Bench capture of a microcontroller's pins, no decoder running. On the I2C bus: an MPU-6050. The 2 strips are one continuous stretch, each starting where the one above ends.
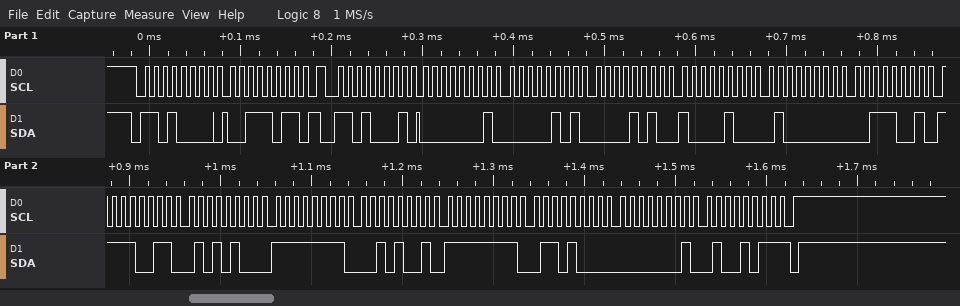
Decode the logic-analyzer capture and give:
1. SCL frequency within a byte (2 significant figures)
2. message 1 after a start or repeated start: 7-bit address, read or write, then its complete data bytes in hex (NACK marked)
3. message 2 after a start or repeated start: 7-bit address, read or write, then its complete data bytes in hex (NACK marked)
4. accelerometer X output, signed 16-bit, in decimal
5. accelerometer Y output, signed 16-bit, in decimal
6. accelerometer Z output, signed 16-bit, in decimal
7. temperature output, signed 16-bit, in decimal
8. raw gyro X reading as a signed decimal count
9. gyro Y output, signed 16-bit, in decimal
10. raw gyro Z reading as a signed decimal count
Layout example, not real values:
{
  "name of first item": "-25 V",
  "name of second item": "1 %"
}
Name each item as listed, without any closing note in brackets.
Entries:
{
  "SCL frequency within a byte": "100 kHz",
  "message 1 after a start or repeated start: 7-bit address, read or write, then its complete data bytes in hex": "0x68 write: 3B",
  "message 2 after a start or repeated start: 7-bit address, read or write, then its complete data bytes in hex": "0x68 read: 01 05 0A 84 40 39 F3 54 FF 29 FF 68 01 4B NACK",
  "accelerometer X output, signed 16-bit, in decimal": "261",
  "accelerometer Y output, signed 16-bit, in decimal": "2692",
  "accelerometer Z output, signed 16-bit, in decimal": "16441",
  "temperature output, signed 16-bit, in decimal": "-3244",
  "raw gyro X reading as a signed decimal count": "-215",
  "gyro Y output, signed 16-bit, in decimal": "-152",
  "raw gyro Z reading as a signed decimal count": "331"
}
